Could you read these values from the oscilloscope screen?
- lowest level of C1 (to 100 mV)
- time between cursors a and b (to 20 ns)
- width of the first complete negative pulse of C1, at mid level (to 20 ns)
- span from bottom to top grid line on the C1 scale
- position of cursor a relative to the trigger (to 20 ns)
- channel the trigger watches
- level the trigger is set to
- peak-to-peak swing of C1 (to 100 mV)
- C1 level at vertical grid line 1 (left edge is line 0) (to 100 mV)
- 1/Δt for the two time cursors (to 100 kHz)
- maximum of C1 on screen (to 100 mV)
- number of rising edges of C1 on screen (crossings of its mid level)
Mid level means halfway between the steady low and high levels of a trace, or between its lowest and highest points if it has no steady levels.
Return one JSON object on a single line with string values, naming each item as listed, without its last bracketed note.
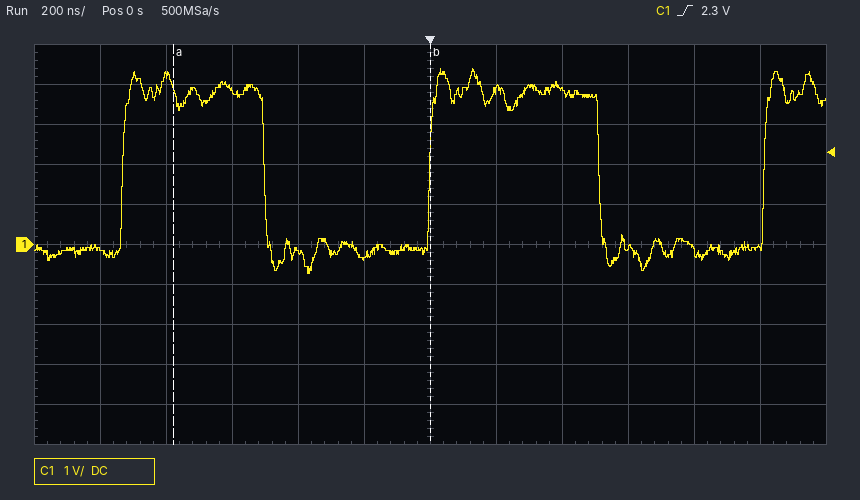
{"lowest level of C1": "-700 mV", "time between cursors a and b": "780 ns", "width of the first complete negative pulse of C1, at mid level": "500 ns", "span from bottom to top grid line on the C1 scale": "10 V", "position of cursor a relative to the trigger": "-780 ns", "channel the trigger watches": "C1", "level the trigger is set to": "2.3 V", "peak-to-peak swing of C1": "5.1 V", "C1 level at vertical grid line 1 (left edge is line 0)": "-100 mV", "1/Δt for the two time cursors": "1.3 MHz", "maximum of C1 on screen": "4.4 V", "number of rising edges of C1 on screen": "3"}
